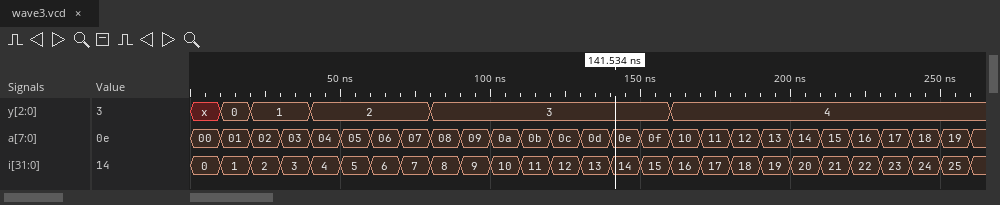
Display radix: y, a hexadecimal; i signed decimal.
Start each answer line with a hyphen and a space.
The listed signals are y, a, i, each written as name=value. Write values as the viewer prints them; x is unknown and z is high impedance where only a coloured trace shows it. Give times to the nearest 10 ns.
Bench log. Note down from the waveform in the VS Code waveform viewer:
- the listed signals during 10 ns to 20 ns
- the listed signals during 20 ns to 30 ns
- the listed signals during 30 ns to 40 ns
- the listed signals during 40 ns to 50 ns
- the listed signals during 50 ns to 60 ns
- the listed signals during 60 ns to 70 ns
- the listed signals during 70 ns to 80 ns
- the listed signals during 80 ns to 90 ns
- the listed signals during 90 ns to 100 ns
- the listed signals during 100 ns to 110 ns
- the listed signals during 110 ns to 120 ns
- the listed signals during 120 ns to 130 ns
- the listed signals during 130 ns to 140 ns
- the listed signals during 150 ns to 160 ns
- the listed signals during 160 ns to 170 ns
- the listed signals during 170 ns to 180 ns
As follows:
- y=0, a=01, i=1
- y=1, a=02, i=2
- y=1, a=03, i=3
- y=2, a=04, i=4
- y=2, a=05, i=5
- y=2, a=06, i=6
- y=2, a=07, i=7
- y=3, a=08, i=8
- y=3, a=09, i=9
- y=3, a=0a, i=10
- y=3, a=0b, i=11
- y=3, a=0c, i=12
- y=3, a=0d, i=13
- y=3, a=0f, i=15
- y=4, a=10, i=16
- y=4, a=11, i=17
